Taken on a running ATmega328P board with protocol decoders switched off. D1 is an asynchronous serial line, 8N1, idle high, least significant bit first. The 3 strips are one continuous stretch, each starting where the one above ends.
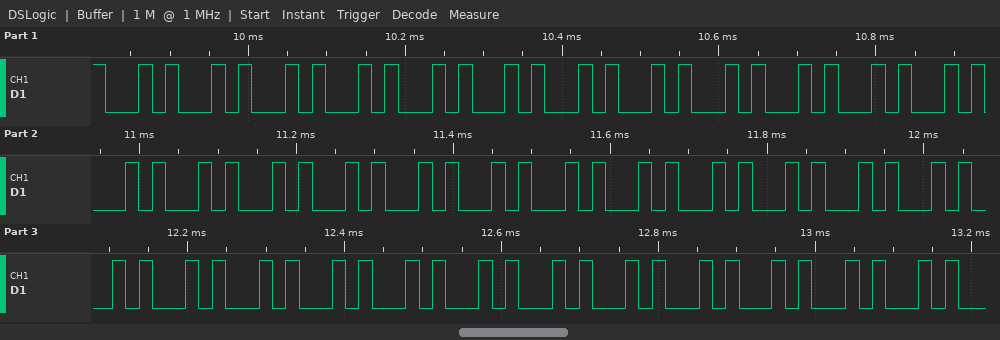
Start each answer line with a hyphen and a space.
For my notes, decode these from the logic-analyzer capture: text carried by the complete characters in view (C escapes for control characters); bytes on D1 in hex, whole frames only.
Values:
- "000000000000000000000000000000000000"
- 30 30 30 30 30 30 30 30 30 30 30 30 30 30 30 30 30 30 30 30 30 30 30 30 30 30 30 30 30 30 30 30 30 30 30 30
